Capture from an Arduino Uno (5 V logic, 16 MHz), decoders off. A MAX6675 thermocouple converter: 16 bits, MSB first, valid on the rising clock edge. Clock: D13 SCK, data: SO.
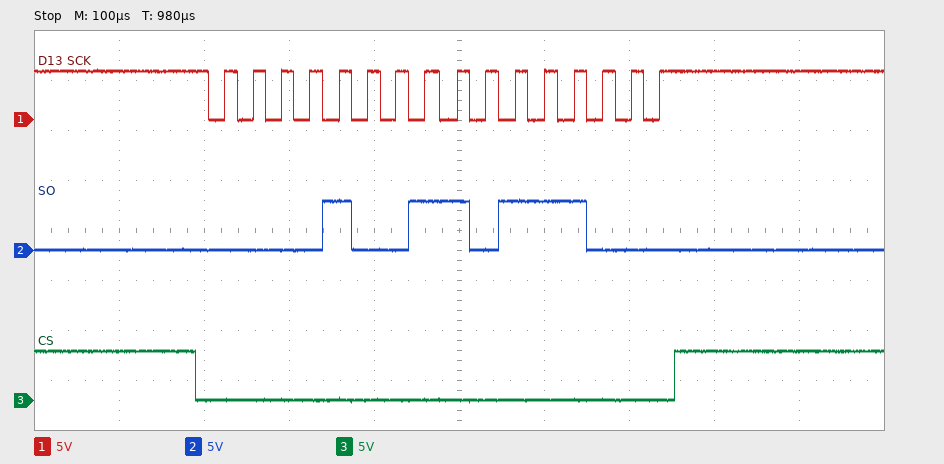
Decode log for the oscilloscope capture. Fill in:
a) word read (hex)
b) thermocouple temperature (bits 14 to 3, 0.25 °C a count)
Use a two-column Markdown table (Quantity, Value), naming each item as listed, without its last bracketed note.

| Quantity | Value |
|---|---|
| word read | 0x09B8 |
| thermocouple temperature | 77.75 °C |
